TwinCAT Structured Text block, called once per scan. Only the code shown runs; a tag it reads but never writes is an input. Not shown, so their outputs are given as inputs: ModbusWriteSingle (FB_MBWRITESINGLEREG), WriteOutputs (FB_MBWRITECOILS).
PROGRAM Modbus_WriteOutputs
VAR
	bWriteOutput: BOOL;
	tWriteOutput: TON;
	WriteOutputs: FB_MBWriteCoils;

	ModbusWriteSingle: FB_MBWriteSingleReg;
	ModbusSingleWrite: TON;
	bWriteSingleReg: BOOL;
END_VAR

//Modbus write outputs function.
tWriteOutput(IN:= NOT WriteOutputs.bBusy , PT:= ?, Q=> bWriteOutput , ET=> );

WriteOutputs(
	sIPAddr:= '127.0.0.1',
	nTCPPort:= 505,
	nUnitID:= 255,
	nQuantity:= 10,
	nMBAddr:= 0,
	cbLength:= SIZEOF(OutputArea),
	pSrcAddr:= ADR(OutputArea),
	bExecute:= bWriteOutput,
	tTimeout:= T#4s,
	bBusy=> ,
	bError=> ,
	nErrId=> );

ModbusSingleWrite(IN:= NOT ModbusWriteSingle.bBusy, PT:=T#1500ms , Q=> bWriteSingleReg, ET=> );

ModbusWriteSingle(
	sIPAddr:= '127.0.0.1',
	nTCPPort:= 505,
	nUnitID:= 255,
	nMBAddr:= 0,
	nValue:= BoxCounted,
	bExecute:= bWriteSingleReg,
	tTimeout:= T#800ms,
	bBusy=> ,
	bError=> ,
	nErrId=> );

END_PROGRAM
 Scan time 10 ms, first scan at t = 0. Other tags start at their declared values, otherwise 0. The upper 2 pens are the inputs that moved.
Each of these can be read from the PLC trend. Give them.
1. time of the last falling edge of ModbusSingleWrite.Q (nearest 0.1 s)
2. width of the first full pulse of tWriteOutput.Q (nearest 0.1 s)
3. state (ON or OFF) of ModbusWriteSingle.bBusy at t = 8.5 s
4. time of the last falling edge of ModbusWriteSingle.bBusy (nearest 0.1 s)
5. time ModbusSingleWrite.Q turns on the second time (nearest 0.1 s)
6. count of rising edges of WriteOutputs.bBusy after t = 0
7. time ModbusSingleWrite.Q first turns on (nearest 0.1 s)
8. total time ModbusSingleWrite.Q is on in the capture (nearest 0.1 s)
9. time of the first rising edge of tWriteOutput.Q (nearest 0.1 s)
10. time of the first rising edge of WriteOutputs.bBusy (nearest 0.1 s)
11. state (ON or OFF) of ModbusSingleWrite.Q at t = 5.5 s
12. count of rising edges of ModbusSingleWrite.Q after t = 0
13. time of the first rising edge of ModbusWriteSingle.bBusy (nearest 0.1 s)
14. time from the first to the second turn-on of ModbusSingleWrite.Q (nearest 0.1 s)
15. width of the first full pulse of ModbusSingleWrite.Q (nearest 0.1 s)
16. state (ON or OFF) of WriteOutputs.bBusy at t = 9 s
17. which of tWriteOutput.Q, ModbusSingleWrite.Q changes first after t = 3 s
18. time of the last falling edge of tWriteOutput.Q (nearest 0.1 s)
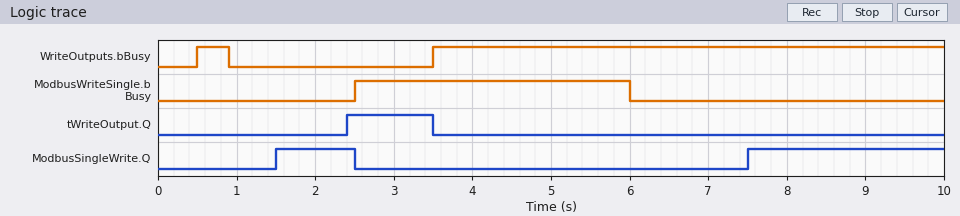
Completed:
2.5 s
1.1 s
OFF
6.0 s
7.5 s
2
1.5 s
3.5 s
2.4 s
0.5 s
OFF
2
2.5 s
6.0 s
1.0 s
ON
tWriteOutput.Q
3.5 s
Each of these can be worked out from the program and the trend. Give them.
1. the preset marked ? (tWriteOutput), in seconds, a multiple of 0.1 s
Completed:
1.5 s
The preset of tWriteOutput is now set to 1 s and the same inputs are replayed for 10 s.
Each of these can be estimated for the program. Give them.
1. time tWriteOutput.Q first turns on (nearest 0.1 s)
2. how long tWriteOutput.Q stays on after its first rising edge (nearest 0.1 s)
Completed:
1.9 s
1.6 s
